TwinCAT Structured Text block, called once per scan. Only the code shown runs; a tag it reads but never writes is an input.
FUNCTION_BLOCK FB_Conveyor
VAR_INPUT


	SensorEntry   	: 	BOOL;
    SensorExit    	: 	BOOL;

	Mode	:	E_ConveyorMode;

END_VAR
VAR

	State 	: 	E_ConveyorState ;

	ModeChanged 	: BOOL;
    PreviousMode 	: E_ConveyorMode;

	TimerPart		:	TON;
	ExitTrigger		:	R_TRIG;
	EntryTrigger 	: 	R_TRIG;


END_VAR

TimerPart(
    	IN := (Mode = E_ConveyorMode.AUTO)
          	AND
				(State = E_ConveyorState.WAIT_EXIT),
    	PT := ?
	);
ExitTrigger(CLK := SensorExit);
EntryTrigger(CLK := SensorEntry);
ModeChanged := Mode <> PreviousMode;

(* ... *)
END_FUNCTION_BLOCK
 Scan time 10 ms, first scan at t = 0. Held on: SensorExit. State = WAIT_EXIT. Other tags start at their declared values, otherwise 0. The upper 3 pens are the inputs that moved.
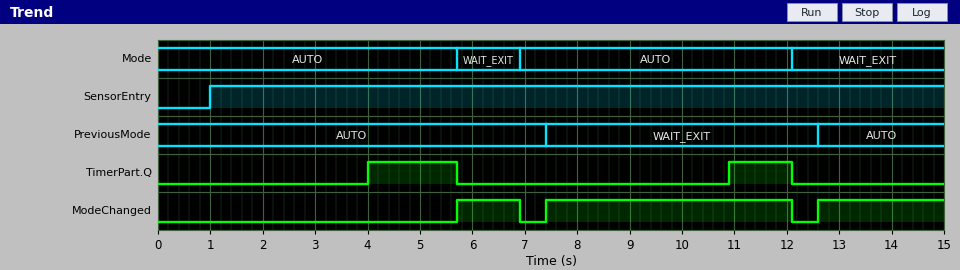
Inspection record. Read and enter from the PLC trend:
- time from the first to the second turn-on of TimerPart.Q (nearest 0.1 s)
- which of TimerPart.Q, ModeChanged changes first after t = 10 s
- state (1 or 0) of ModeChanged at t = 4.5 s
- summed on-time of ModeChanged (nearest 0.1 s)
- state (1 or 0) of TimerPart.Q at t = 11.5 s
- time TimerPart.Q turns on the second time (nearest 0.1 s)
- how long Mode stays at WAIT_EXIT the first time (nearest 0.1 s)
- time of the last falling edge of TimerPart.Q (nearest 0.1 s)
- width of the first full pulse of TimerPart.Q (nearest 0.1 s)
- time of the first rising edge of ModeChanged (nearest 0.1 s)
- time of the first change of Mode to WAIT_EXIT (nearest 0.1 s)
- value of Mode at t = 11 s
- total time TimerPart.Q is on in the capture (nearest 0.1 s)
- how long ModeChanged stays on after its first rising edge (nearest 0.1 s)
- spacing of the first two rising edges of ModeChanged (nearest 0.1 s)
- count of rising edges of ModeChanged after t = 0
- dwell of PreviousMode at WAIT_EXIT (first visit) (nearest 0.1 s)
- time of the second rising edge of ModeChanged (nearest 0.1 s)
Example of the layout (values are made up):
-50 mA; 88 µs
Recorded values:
6.9 s; TimerPart.Q; 0; 8.3 s; 1; 10.9 s; 1.2 s; 12.1 s; 1.7 s; 5.7 s; 5.7 s; AUTO; 2.9 s; 1.2 s; 1.7 s; 3; 5.2 s; 7.4 s
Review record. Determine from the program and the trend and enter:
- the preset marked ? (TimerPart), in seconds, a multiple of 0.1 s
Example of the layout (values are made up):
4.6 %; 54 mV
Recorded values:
4.0 s
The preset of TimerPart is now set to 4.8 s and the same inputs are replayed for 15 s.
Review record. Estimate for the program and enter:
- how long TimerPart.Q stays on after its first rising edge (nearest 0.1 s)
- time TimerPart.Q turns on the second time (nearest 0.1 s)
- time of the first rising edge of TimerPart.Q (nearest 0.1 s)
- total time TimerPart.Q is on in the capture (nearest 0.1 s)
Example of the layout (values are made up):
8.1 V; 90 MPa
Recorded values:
0.9 s; 11.7 s; 4.8 s; 1.3 s
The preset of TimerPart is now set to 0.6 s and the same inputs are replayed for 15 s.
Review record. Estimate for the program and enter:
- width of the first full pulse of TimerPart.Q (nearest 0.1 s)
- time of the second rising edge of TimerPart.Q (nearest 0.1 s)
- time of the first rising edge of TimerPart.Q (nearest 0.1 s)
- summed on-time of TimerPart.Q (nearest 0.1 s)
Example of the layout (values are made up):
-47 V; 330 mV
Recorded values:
5.1 s; 7.5 s; 0.6 s; 9.7 s
